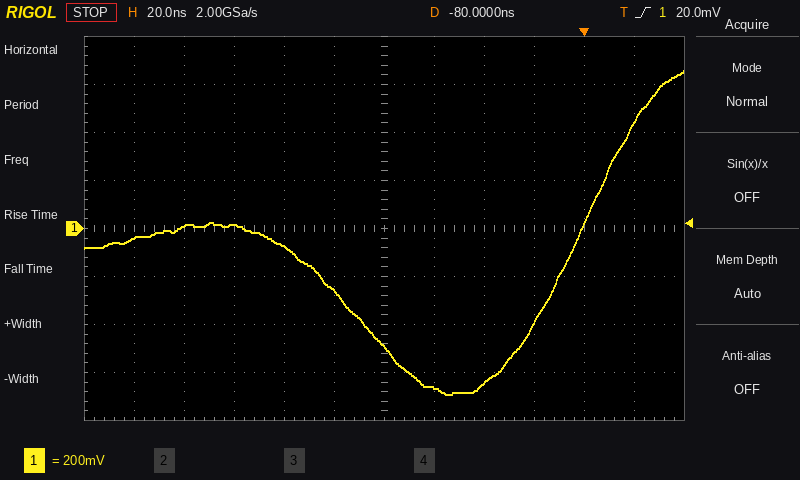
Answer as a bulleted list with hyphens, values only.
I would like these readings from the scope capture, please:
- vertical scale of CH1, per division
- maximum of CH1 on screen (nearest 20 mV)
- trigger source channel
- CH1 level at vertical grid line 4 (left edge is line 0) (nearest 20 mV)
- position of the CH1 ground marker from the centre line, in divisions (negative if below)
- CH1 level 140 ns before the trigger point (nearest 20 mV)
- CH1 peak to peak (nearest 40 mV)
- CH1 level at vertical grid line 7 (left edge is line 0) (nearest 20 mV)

- 200 mV
- 660 mV
- CH1
- -80 mV
- 0.0 div
- 20 mV
- 1.36 V
- -660 mV
